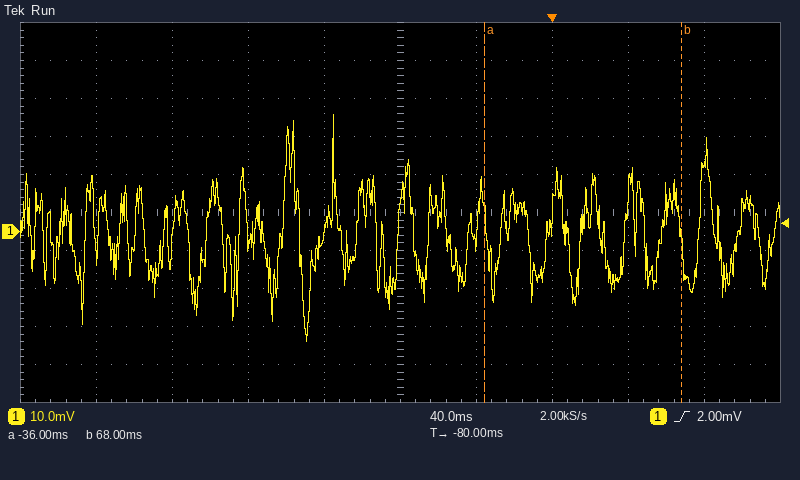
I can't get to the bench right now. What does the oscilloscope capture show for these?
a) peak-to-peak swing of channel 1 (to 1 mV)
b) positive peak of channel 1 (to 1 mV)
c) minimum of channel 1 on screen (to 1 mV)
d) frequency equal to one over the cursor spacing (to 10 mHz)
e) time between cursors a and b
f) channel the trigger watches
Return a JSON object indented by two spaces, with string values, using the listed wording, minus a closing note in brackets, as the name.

{
  "peak-to-peak swing of channel 1": "60 mV",
  "positive peak of channel 1": "31 mV",
  "minimum of channel 1 on screen": "-29 mV",
  "frequency equal to one over the cursor spacing": "9.62 Hz",
  "time between cursors a and b": "104 ms",
  "channel the trigger watches": "channel 1"
}
